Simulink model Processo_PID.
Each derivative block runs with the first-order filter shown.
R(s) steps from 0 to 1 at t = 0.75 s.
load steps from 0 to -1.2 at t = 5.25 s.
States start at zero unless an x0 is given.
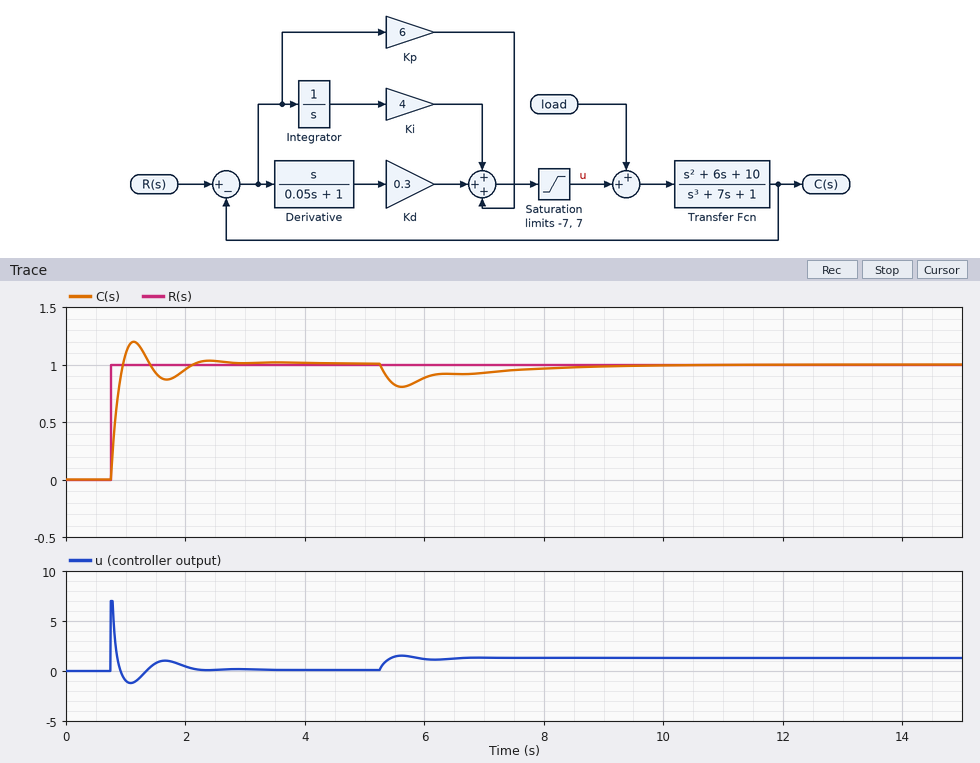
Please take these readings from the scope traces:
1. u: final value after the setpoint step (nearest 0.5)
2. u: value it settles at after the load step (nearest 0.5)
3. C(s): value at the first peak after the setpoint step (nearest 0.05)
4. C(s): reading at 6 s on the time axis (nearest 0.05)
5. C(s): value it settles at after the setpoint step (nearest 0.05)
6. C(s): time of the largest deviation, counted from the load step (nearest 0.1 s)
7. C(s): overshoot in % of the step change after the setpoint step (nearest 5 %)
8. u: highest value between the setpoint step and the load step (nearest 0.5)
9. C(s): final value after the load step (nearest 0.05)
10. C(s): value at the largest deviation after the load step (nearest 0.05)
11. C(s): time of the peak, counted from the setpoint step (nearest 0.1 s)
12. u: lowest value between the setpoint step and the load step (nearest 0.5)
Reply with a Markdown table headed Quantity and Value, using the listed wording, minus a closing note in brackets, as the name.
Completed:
| Quantity | Value |
|---|---|
| u: final value after the setpoint step | 0.0 |
| u: value it settles at after the load step | 1.5 |
| C(s): value at the first peak after the setpoint step | 1.20 |
| C(s): reading at 6 s on the time axis | 0.90 |
| C(s): value it settles at after the setpoint step | 1.00 |
| C(s): time of the largest deviation, counted from the load step | 0.4 s |
| C(s): overshoot in % of the step change after the setpoint step | 20 % |
| u: highest value between the setpoint step and the load step | 7.0 |
| C(s): final value after the load step | 1.00 |
| C(s): value at the largest deviation after the load step | 0.80 |
| C(s): time of the peak, counted from the setpoint step | 0.4 s |
| u: lowest value between the setpoint step and the load step | -1.0 |
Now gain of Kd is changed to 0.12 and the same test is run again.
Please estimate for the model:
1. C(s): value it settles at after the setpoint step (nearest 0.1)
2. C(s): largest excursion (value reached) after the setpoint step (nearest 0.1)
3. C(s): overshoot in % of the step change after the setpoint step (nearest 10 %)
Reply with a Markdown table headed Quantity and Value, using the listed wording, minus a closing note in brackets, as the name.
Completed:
| Quantity | Value |
|---|---|
| C(s): value it settles at after the setpoint step | 1.0 |
| C(s): largest excursion (value reached) after the setpoint step | 1.3 |
| C(s): overshoot in % of the step change after the setpoint step | 30 % |
